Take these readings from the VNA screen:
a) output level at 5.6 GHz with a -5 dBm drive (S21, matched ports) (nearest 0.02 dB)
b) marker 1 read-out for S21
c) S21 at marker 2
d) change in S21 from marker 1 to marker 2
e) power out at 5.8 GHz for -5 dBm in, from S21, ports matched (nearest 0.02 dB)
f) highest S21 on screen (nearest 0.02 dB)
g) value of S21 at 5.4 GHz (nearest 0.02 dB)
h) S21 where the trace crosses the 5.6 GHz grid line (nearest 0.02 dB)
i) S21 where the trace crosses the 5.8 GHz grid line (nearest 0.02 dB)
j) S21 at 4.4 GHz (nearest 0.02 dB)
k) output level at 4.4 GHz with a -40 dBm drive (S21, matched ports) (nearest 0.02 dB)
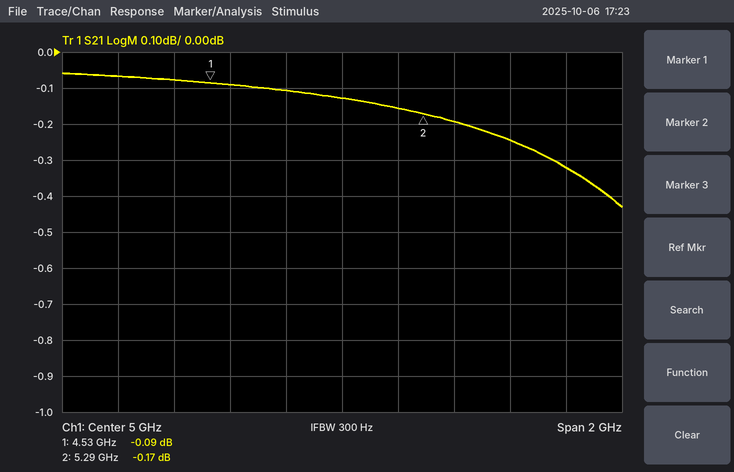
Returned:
-5.24 dBm
-0.09 dB
-0.17 dB
-0.08 dB
-5.32 dBm
-0.06 dB
-0.20 dB
-0.24 dB
-0.32 dB
-0.08 dB
-40.08 dBm
